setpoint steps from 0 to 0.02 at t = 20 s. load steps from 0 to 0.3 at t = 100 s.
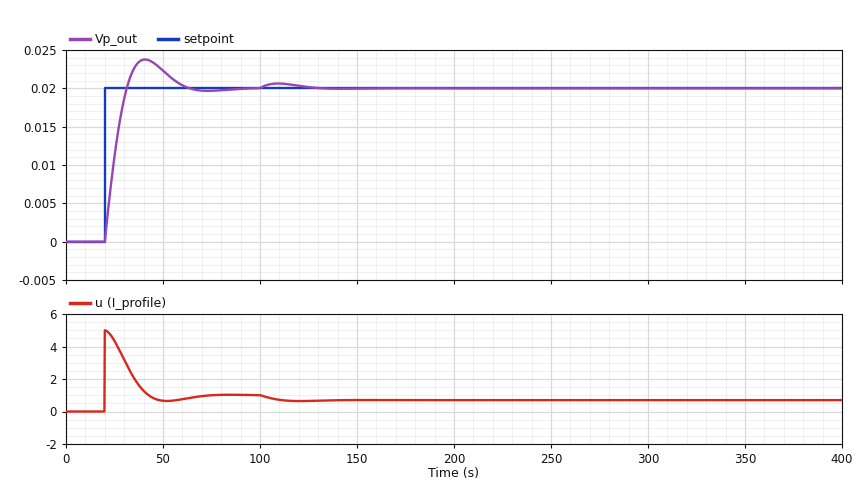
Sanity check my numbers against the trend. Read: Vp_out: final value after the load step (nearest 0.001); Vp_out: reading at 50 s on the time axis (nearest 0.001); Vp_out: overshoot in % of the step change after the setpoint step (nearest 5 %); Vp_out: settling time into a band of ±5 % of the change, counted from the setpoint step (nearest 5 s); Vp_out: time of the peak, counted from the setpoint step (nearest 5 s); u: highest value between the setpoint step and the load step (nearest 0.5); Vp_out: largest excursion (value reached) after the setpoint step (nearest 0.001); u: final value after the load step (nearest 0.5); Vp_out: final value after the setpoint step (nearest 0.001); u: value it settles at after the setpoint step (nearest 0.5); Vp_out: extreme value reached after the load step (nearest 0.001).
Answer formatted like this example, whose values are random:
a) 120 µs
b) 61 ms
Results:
a) 0.020
b) 0.022
c) 20 %
d) 35 s
e) 20 s
f) 5.0
g) 0.024
h) 0.5
i) 0.020
j) 1.0
k) 0.021
